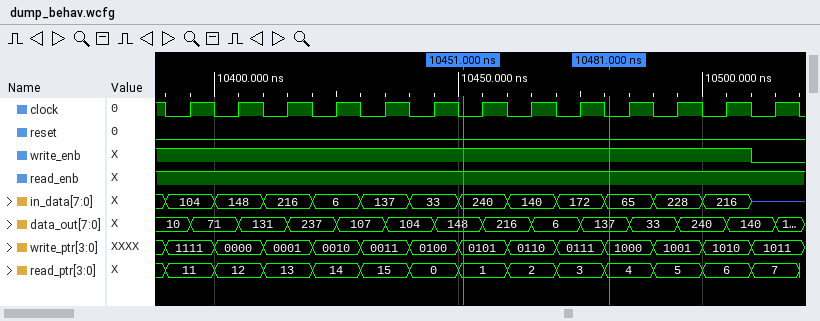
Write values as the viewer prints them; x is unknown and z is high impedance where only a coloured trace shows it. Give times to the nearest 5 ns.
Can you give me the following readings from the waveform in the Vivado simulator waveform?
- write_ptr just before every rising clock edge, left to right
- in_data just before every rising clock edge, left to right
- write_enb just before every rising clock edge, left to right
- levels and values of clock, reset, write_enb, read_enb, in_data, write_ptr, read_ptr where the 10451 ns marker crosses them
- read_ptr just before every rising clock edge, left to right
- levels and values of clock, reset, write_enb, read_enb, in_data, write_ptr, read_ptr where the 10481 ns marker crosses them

1111, 0000, 0001, 0010, 0011, 0100, 0101, 0110, 0111, 1000, 1001, 1010, 1011
104, 148, 216, 6, 137, 33, 240, 140, 172, 65, 228, 216, z
1 1 1 1 1 1 1 1 1 1 1 1 0
clock=0, reset=0, write_enb=1, read_enb=1, in_data=240, write_ptr=0101, read_ptr=1
11, 12, 13, 14, 15, 0, 1, 2, 3, 4, 5, 6, 7
clock=0, reset=0, write_enb=1, read_enb=1, in_data=65, write_ptr=1000, read_ptr=4
